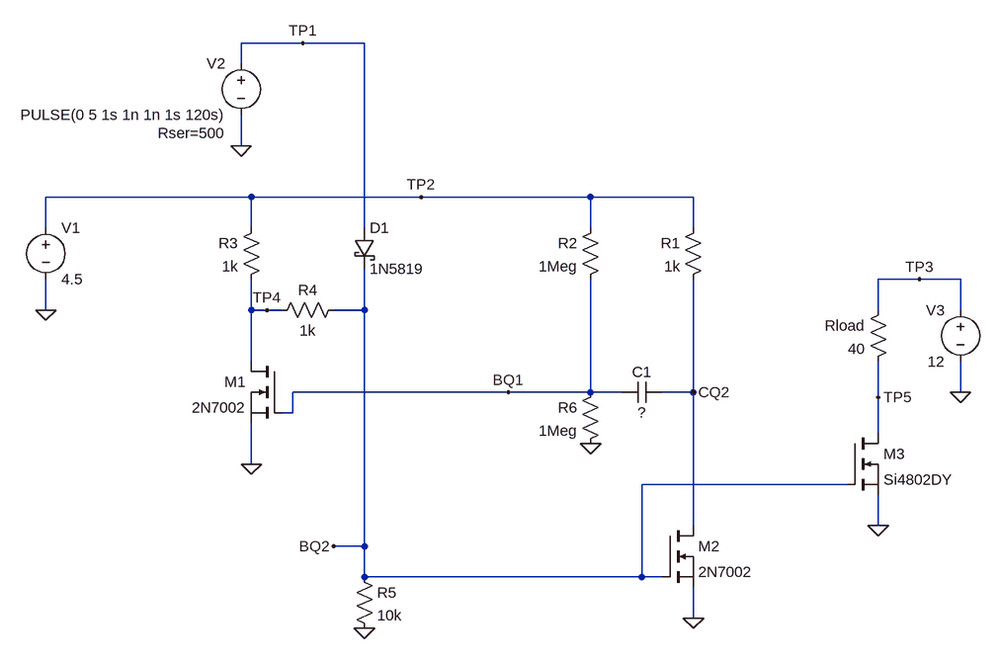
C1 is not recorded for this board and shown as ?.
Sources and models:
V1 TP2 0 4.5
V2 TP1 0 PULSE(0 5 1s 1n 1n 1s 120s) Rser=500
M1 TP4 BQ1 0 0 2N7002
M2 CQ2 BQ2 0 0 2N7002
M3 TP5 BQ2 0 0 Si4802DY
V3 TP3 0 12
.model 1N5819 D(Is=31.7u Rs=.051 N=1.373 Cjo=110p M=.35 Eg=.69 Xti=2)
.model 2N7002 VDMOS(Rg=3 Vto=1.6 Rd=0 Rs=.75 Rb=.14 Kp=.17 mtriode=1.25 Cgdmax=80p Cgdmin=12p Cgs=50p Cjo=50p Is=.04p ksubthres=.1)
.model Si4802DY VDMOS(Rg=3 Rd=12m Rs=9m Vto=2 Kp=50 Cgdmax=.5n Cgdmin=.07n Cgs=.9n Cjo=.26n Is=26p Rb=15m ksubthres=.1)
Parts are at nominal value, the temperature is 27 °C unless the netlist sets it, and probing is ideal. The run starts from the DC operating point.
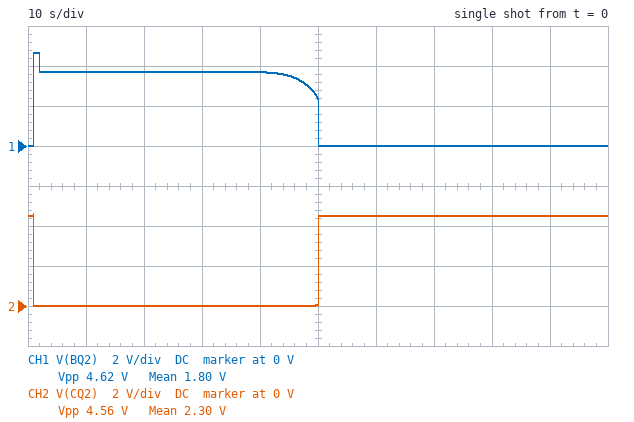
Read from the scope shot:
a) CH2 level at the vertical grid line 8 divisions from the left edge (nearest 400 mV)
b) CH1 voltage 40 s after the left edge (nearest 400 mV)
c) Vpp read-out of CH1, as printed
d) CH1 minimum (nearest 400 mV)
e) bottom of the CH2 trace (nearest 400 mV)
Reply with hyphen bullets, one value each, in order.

- 4.4 V
- 3.6 V
- 4.62 V
- 0 V
- 0 V
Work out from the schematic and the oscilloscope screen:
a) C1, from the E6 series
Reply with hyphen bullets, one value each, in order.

- 47 µF
